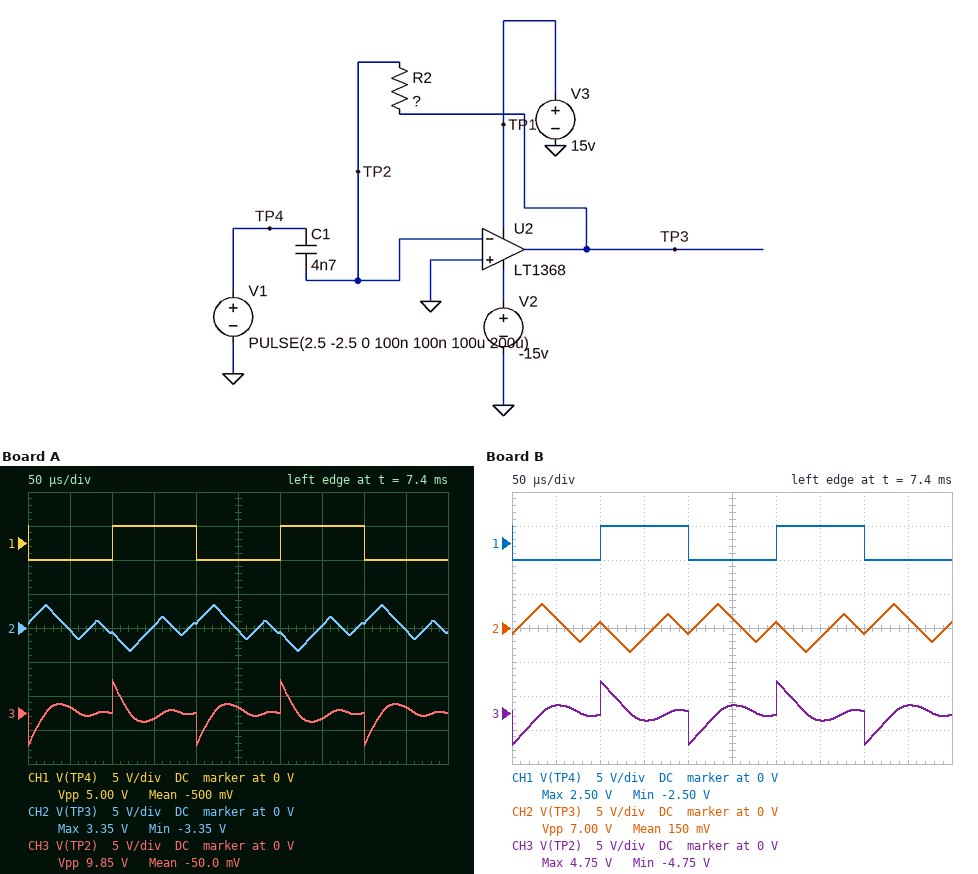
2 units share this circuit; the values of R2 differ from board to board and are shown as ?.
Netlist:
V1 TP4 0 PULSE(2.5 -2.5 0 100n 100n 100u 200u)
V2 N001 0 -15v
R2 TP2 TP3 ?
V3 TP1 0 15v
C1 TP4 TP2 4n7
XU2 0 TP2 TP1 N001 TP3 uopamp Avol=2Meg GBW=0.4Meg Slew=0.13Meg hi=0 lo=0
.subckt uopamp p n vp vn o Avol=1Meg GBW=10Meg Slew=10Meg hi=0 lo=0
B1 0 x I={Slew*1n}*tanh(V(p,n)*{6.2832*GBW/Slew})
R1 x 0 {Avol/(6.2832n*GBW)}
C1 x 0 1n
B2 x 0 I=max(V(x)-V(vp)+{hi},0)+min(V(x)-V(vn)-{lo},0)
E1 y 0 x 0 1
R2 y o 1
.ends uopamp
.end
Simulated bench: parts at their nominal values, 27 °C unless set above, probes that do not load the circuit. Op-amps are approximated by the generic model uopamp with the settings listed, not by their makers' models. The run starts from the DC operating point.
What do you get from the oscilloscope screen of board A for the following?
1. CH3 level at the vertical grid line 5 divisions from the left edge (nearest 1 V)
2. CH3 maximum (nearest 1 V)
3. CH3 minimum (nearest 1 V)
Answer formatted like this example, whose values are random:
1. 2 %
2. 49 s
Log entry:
1. 1 V
2. 5 V
3. -5 V
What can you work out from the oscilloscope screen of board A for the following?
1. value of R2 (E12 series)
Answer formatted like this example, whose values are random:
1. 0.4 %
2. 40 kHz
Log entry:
1. 3.9 kΩ
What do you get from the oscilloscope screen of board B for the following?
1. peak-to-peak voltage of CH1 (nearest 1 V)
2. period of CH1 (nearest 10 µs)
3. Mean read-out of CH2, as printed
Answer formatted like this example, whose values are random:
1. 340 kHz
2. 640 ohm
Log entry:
1. 5 V
2. 200 µs
3. 150 mV
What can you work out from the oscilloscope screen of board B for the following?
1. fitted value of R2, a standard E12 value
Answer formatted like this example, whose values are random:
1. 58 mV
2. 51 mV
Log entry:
1. 5.6 kΩ
